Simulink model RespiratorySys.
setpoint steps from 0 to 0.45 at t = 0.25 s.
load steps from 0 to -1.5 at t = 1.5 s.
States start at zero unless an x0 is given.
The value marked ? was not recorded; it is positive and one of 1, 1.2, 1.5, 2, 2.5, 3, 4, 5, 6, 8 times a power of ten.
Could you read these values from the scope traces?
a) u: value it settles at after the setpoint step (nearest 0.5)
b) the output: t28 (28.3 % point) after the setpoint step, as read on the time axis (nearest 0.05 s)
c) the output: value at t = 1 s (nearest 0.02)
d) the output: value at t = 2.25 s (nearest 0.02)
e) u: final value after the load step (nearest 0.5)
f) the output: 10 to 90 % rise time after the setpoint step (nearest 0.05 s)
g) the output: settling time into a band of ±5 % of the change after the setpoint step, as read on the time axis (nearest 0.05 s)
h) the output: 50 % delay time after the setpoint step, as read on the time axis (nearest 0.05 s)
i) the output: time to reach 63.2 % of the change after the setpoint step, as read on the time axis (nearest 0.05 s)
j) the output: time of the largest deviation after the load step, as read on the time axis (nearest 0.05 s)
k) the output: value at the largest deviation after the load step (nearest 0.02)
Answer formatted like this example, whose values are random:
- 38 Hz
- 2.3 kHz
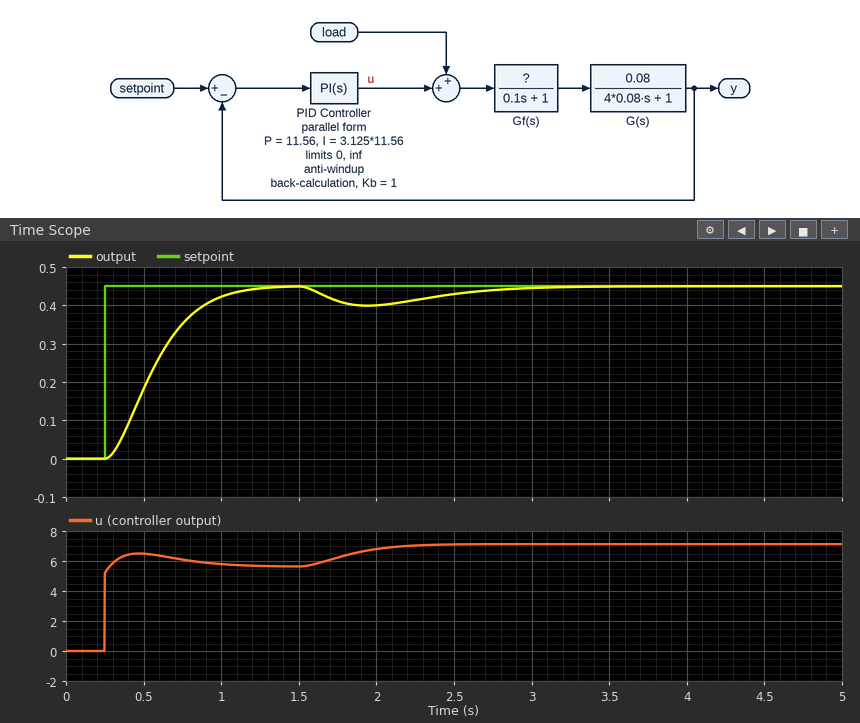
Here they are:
- 5.5
- 0.45 s
- 0.42
- 0.42
- 7.0
- 0.55 s
- 1.05 s
- 0.55 s
- 0.65 s
- 1.95 s
- 0.40
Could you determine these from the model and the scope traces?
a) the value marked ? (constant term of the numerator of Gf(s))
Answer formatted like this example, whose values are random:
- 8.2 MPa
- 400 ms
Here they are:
- 1
